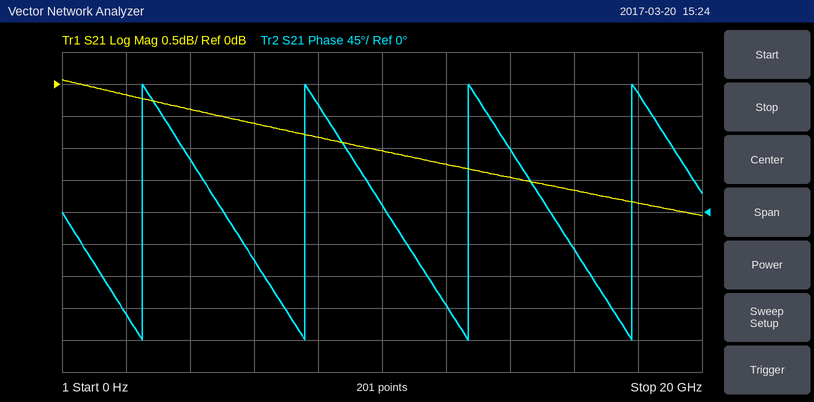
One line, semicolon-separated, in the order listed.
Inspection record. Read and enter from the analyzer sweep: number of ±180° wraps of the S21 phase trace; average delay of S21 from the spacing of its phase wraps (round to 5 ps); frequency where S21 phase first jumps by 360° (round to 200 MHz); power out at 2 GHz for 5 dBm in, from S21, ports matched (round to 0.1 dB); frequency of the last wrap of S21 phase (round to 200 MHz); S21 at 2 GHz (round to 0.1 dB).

4; 195 ps; 2.6 GHz; 4.8 dBm; 17.8 GHz; -0.2 dB
